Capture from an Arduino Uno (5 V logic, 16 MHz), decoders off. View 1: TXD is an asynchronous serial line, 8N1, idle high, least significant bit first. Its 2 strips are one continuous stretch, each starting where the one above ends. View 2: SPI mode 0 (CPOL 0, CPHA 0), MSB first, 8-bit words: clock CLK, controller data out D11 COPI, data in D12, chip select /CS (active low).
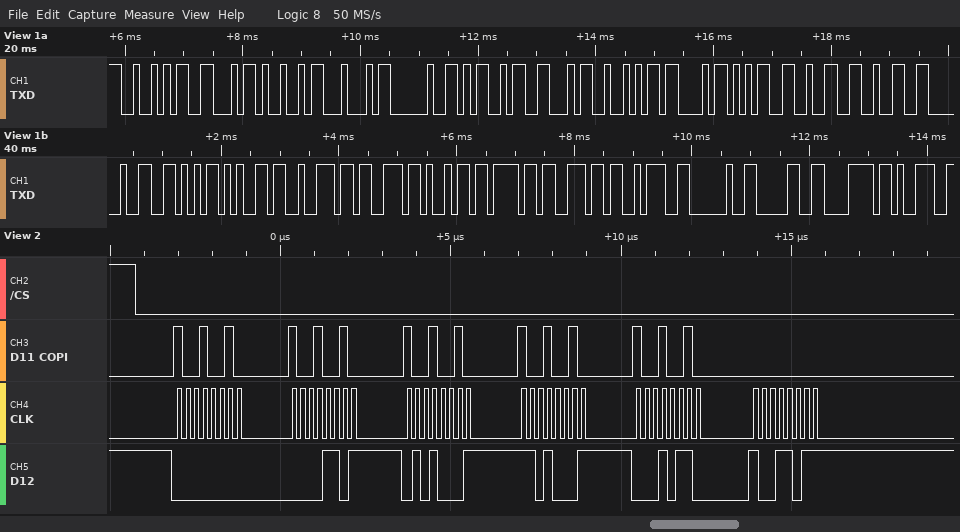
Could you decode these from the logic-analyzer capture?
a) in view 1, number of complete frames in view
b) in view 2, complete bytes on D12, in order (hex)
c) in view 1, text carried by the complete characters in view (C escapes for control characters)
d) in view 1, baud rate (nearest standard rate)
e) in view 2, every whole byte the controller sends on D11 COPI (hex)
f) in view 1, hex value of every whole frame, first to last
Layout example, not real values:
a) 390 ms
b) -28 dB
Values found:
a) 25
b) 00 0D 51 D1 16 9B
c) "RFID MFRC522 Version: 0x9"
d) 9600 baud
e) 92 92 92 92 92 00
f) 0x52 0x46 0x49 0x44 0x20 0x4D 0x46 0x52 0x43 0x35 0x32 0x32 0x20 0x56 0x65 0x72 0x73 0x69 0x6F 0x6E 0x3A 0x20 0x30 0x78 0x39
